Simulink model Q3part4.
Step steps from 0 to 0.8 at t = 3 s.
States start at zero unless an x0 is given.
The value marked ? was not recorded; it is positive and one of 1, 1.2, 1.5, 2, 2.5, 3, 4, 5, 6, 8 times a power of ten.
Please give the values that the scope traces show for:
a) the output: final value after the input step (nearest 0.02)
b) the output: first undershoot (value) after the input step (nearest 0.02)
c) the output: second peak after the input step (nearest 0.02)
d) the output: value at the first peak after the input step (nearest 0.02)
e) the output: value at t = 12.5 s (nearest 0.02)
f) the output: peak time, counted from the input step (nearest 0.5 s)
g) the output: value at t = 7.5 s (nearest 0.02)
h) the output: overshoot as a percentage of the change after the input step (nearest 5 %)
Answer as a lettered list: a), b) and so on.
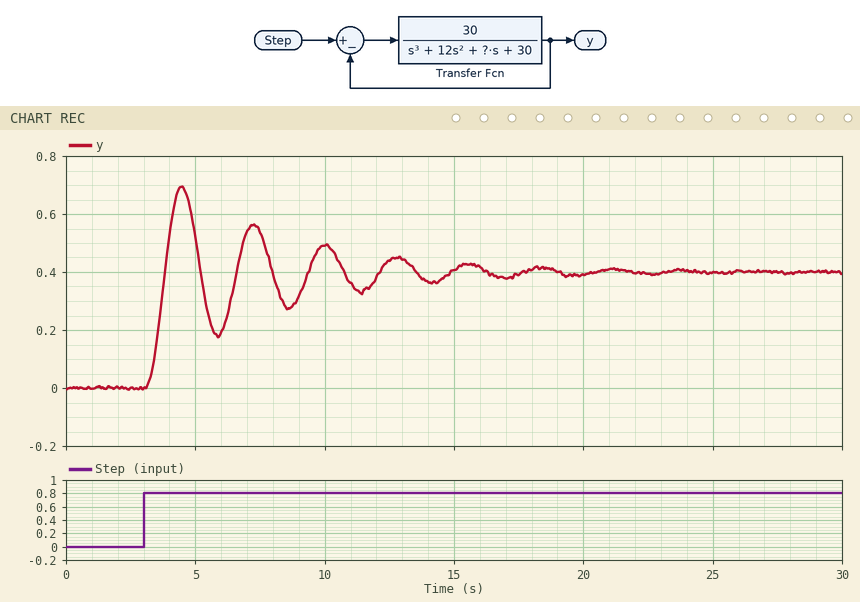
a) 0.40
b) 0.18
c) 0.56
d) 0.70
e) 0.44
f) 1.5 s
g) 0.54
h) 75 %
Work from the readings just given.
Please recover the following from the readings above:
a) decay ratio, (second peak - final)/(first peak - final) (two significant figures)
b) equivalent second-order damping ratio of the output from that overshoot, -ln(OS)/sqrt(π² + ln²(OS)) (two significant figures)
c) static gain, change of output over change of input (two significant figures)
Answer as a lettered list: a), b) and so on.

a) 0.53
b) 0.091
c) 0.50
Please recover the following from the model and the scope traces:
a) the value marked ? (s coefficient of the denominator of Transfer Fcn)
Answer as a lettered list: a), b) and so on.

a) 10
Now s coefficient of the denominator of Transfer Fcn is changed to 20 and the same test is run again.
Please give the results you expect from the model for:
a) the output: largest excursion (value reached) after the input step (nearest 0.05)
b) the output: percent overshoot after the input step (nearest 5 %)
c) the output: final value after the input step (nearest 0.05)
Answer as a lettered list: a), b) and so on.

a) 0.55
b) 40 %
c) 0.40
